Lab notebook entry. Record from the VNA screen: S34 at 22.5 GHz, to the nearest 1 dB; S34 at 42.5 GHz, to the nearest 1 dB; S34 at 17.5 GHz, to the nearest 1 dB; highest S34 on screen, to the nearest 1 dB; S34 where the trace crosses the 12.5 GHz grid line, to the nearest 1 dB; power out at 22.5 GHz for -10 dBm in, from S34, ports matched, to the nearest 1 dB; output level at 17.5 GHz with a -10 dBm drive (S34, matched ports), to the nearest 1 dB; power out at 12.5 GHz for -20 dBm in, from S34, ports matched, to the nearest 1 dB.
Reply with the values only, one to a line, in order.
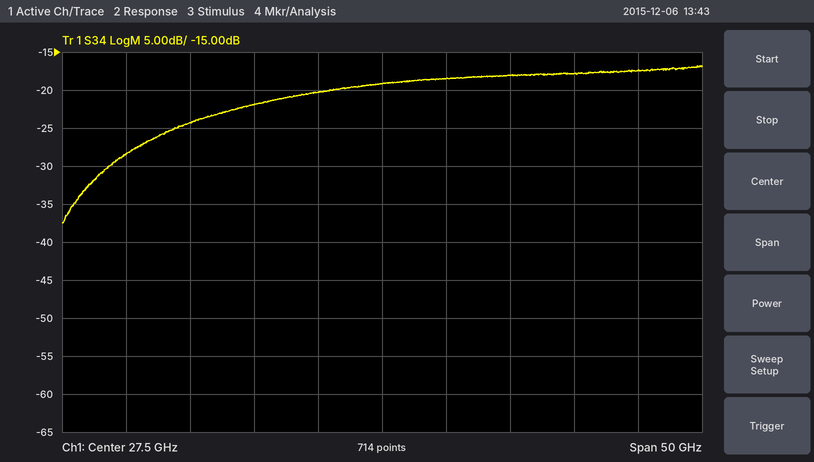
-20 dB
-18 dB
-22 dB
-17 dB
-24 dB
-30 dBm
-32 dBm
-44 dBm
